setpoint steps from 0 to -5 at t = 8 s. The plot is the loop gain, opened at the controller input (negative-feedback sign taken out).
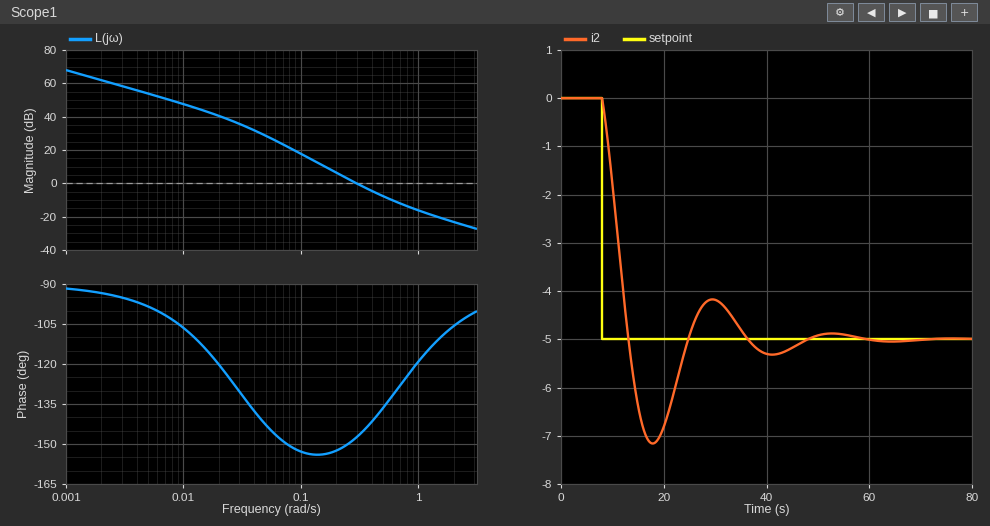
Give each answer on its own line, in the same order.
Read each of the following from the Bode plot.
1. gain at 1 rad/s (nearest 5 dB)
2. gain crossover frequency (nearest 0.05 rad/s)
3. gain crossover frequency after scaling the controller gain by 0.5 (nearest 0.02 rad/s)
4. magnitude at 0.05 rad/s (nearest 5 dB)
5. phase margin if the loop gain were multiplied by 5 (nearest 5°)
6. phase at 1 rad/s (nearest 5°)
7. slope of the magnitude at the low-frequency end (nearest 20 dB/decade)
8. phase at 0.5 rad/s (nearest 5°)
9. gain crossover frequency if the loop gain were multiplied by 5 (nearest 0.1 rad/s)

-15 dB
0.30 rad/s
0.20 rad/s
30 dB
55°
-120°
-20 dB/decade
-135°
0.8 rad/s
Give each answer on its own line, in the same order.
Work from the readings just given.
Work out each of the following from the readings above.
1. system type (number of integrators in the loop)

1
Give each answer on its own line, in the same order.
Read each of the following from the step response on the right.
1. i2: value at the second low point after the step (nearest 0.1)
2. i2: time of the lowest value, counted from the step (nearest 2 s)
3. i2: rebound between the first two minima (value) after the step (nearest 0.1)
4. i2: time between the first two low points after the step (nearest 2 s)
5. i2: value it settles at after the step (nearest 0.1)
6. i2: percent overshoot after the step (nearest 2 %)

-5.3
10 s
-4.2
24 s
-5.0
44 %
